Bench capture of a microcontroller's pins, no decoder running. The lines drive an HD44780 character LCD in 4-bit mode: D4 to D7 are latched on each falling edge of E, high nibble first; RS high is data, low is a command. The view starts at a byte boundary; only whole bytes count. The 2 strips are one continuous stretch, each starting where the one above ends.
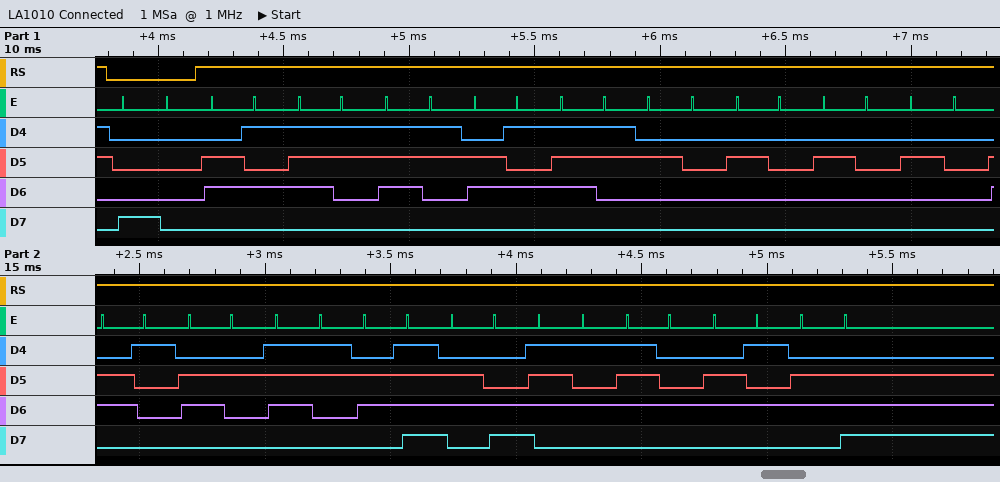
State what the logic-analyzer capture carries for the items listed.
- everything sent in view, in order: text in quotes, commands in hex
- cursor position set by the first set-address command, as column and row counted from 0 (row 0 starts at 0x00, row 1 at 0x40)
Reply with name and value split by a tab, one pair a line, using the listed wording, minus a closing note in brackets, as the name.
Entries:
everything sent in view, in order: text in quotes, commands in hex	0x80 "esses    absoluten"
cursor position set by the first set-address command, as column and row counted from 0	column 0, row 0
